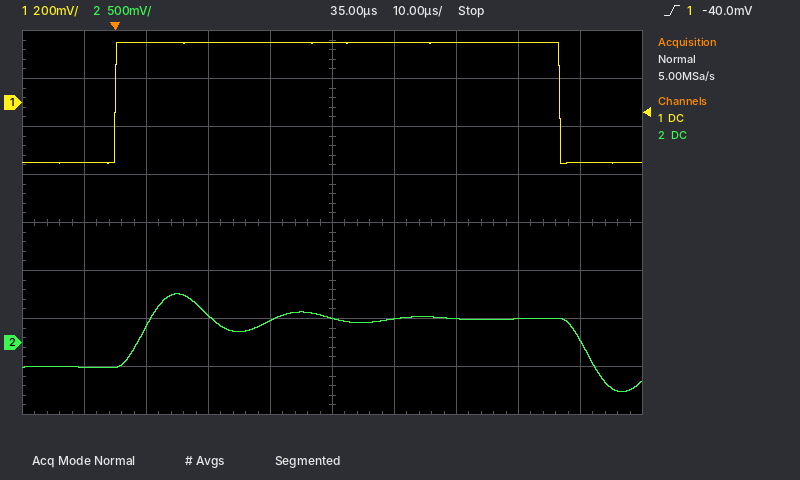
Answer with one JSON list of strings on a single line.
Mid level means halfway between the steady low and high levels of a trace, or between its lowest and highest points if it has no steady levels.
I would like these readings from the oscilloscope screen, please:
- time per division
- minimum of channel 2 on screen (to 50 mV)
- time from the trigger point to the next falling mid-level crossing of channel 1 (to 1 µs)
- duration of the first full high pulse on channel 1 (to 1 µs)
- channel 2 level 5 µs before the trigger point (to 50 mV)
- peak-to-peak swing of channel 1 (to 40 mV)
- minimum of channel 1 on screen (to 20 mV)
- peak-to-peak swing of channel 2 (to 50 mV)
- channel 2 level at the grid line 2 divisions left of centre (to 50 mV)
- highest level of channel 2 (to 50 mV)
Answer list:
["10 µs", "-500 mV", "72 µs", "72 µs", "-250 mV", "520 mV", "-260 mV", "1.00 V", "300 mV", "500 mV"]
